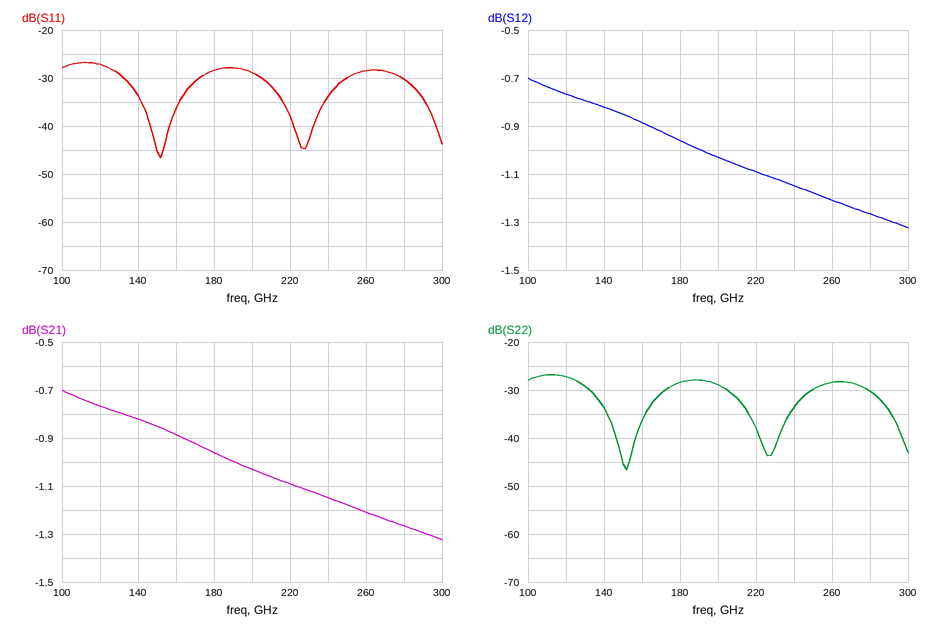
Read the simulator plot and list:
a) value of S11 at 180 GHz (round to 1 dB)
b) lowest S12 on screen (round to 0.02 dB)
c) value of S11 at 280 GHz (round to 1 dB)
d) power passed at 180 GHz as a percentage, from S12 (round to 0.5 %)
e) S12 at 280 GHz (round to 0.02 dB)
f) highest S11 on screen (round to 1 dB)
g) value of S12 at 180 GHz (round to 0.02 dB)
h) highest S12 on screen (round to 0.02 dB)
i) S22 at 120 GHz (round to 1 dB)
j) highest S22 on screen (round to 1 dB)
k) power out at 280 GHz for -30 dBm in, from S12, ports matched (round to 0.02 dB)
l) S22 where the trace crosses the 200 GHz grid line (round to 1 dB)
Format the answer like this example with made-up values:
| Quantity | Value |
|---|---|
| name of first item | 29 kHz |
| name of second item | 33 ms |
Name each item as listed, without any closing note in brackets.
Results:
| Quantity | Value |
|---|---|
| value of S11 at 180 GHz | -28 dB |
| lowest S12 on screen | -1.32 dB |
| value of S11 at 280 GHz | -30 dB |
| power passed at 180 GHz as a percentage, from S12 | 80.0 % |
| S12 at 280 GHz | -1.26 dB |
| highest S11 on screen | -27 dB |
| value of S12 at 180 GHz | -0.96 dB |
| highest S12 on screen | -0.70 dB |
| S22 at 120 GHz | -27 dB |
| highest S22 on screen | -27 dB |
| power out at 280 GHz for -30 dBm in, from S12, ports matched | -31.26 dBm |
| S22 where the trace crosses the 200 GHz grid line | -29 dB |
